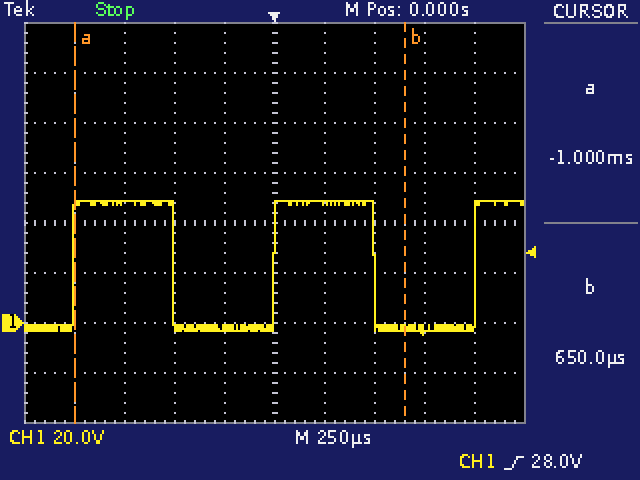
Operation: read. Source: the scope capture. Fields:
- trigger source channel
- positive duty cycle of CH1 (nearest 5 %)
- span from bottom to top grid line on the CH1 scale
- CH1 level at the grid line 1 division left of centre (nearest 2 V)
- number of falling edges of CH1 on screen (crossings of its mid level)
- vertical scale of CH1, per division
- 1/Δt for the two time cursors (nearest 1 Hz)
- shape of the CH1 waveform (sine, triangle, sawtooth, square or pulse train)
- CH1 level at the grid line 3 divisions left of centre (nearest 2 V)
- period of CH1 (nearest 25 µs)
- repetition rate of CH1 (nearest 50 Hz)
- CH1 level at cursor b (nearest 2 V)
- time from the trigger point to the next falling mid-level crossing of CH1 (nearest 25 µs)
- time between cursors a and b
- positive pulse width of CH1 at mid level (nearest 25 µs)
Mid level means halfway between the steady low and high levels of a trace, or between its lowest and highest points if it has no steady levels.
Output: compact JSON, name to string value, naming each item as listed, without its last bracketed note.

{"trigger source channel": "CH1", "positive duty cycle of CH1": "50 %", "span from bottom to top grid line on the CH1 scale": "160 V", "CH1 level at the grid line 1 division left of centre": "-2 V", "number of falling edges of CH1 on screen": "2", "vertical scale of CH1, per division": "20 V", "1/Δt for the two time cursors": "606 Hz", "shape of the CH1 waveform": "square", "CH1 level at the grid line 3 divisions left of centre": "48 V", "period of CH1": "1.000 ms", "repetition rate of CH1": "1.00 kHz", "CH1 level at cursor b": "-2 V", "time from the trigger point to the next falling mid-level crossing of CH1": "500 µs", "time between cursors a and b": "1.650 ms", "positive pulse width of CH1 at mid level": "500 µs"}
